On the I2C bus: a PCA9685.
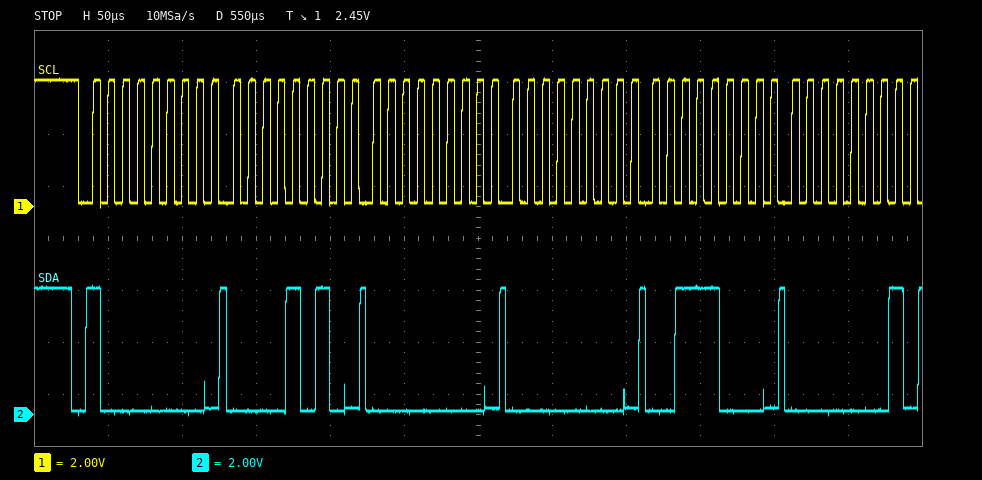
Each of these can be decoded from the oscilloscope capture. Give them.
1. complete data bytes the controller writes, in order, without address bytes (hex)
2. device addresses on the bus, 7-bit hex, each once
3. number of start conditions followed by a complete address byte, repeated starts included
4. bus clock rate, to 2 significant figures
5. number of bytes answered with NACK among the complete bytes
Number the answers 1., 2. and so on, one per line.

1. 0A 00 00 38 01
2. 0x40
3. 1
4. 100 kHz
5. 0
